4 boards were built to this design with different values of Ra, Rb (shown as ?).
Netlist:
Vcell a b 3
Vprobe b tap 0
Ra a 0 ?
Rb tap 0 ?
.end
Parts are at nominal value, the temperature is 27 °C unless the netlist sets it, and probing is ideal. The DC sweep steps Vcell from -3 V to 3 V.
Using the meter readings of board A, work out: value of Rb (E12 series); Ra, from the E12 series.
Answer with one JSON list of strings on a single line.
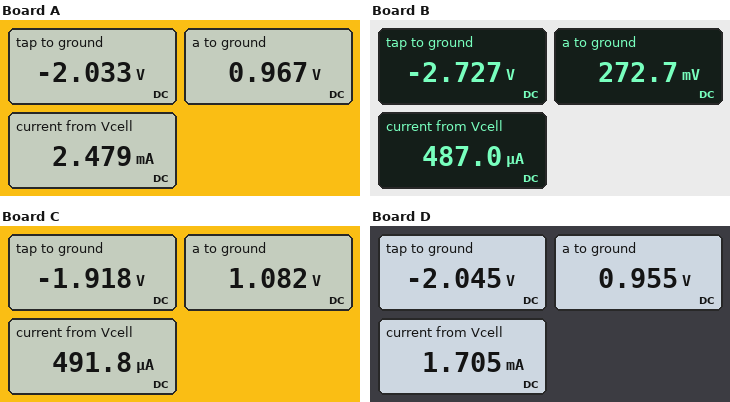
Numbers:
["820 Ω", "390 Ω"]
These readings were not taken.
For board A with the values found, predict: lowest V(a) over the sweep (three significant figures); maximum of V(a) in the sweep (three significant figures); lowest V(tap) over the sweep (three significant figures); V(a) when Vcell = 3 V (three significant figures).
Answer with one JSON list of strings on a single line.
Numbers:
["-967 mV", "967 mV", "-2.03 V", "967 mV"]
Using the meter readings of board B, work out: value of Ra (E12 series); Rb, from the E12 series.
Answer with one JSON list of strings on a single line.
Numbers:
["560 Ω", "5.6 kΩ"]
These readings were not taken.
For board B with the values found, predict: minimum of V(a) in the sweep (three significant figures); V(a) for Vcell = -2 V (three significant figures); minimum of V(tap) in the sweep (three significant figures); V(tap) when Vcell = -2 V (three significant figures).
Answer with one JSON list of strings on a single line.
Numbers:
["-273 mV", "-182 mV", "-2.73 V", "1.82 V"]
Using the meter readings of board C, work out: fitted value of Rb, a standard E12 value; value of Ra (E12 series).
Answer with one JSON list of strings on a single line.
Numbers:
["3.9 kΩ", "2.2 kΩ"]
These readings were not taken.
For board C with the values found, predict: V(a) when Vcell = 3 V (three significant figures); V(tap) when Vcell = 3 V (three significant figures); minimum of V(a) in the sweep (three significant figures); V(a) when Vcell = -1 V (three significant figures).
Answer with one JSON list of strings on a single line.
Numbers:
["1.08 V", "-1.92 V", "-1.08 V", "-361 mV"]
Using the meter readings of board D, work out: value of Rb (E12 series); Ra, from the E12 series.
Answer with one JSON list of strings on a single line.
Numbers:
["1.2 kΩ", "560 Ω"]
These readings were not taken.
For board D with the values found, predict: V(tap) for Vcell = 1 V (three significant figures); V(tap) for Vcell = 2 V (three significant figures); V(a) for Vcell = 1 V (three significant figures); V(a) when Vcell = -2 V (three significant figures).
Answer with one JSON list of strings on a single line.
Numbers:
["-682 mV", "-1.36 V", "318 mV", "-636 mV"]
